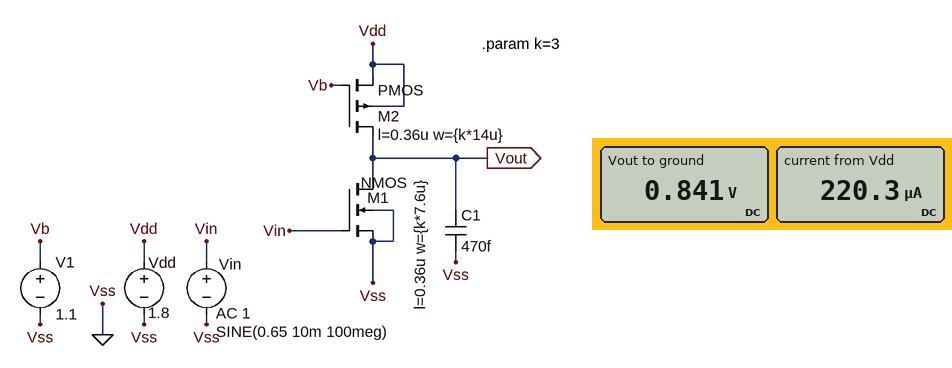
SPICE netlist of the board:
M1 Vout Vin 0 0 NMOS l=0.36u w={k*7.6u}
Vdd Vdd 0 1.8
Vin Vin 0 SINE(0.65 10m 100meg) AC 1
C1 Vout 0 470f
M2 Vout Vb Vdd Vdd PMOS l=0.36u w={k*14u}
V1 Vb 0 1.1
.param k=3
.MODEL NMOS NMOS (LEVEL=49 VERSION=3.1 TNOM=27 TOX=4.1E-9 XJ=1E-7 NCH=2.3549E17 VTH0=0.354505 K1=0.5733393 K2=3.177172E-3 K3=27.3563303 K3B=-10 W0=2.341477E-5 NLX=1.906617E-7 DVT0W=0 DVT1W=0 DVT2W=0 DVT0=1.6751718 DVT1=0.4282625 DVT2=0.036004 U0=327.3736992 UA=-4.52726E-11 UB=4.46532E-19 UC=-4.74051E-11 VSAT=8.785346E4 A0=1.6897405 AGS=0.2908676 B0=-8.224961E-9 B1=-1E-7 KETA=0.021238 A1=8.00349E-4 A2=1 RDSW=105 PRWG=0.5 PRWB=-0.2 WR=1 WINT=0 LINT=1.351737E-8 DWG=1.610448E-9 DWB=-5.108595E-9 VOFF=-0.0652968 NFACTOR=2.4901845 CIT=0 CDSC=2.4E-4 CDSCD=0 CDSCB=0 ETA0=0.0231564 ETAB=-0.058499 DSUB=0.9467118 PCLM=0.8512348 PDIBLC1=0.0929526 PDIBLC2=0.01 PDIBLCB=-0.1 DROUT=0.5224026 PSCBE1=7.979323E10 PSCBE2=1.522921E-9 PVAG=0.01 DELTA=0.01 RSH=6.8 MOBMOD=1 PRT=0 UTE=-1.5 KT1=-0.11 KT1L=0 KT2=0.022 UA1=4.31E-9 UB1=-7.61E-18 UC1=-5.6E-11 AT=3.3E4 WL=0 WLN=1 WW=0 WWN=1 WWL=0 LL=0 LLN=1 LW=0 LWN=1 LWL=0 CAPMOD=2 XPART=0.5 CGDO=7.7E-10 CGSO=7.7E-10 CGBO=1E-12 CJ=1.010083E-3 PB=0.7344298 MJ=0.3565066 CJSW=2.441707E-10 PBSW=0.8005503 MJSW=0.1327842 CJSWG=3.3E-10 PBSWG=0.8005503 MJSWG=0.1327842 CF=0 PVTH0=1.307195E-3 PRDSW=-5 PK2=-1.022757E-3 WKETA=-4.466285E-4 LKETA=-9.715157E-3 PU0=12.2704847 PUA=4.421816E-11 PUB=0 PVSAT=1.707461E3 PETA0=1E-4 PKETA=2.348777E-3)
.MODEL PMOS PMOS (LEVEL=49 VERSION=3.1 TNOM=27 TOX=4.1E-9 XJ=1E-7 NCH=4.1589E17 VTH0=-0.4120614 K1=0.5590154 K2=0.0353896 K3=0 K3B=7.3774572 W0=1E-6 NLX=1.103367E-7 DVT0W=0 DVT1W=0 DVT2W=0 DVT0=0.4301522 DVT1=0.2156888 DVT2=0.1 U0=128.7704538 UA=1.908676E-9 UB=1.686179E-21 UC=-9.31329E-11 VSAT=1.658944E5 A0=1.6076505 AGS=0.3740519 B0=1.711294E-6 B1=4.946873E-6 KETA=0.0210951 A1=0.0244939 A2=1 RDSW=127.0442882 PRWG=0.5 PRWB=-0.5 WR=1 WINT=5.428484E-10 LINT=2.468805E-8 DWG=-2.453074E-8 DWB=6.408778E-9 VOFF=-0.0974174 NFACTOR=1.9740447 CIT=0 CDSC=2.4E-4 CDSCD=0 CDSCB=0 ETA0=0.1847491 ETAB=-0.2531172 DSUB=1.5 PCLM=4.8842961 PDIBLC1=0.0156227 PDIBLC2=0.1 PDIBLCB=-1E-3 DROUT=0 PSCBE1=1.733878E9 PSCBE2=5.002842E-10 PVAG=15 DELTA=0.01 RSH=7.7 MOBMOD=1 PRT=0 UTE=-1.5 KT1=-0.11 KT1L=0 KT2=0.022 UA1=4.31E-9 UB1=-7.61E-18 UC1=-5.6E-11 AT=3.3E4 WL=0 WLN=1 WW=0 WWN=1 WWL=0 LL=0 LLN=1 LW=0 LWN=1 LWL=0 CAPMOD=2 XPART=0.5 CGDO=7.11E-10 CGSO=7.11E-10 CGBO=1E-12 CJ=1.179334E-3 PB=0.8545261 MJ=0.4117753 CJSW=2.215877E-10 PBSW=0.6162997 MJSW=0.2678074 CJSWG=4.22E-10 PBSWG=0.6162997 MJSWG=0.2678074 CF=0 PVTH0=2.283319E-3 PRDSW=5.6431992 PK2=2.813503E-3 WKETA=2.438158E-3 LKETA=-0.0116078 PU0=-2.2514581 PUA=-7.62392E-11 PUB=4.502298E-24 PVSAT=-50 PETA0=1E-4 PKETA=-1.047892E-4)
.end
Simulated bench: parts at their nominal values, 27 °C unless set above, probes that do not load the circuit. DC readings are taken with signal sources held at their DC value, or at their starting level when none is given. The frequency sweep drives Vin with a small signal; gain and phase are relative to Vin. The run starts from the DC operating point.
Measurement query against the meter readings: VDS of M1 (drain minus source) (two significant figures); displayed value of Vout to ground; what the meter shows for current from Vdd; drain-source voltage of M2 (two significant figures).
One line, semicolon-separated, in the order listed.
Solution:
840 mV; 0.841 V; 220.3 µA; -960 mV
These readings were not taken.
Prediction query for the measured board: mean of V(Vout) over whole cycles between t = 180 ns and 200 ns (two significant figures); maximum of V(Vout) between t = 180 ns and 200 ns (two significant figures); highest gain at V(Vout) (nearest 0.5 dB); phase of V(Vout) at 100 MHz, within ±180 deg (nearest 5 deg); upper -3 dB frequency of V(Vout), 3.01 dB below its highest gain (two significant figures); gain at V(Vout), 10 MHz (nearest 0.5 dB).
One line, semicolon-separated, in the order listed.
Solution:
830 mV; 910 mV; 36.0 dB; 95 deg; 13 MHz; 33.5 dB
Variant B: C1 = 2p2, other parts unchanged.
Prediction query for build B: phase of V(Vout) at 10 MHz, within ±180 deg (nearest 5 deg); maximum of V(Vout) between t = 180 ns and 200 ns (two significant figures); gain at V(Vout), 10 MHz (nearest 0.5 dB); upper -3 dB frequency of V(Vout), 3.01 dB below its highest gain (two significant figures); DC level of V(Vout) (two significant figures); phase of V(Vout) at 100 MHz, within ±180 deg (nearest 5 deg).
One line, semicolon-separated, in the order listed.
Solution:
105 deg; 850 mV; 25.0 dB; 3.0 MHz; 840 mV; 90 deg
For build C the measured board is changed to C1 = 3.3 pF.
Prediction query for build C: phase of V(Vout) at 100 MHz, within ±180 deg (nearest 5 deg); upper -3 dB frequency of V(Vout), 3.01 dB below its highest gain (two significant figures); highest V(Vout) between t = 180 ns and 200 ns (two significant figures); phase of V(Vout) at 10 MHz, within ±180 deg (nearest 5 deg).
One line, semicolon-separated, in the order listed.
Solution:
90 deg; 2.0 MHz; 840 mV; 100 deg
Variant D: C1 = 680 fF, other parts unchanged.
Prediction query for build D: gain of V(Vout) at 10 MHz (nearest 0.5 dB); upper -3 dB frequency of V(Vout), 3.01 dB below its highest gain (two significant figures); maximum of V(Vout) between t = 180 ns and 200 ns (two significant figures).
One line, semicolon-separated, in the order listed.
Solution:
32.5 dB; 9.1 MHz; 890 mV
